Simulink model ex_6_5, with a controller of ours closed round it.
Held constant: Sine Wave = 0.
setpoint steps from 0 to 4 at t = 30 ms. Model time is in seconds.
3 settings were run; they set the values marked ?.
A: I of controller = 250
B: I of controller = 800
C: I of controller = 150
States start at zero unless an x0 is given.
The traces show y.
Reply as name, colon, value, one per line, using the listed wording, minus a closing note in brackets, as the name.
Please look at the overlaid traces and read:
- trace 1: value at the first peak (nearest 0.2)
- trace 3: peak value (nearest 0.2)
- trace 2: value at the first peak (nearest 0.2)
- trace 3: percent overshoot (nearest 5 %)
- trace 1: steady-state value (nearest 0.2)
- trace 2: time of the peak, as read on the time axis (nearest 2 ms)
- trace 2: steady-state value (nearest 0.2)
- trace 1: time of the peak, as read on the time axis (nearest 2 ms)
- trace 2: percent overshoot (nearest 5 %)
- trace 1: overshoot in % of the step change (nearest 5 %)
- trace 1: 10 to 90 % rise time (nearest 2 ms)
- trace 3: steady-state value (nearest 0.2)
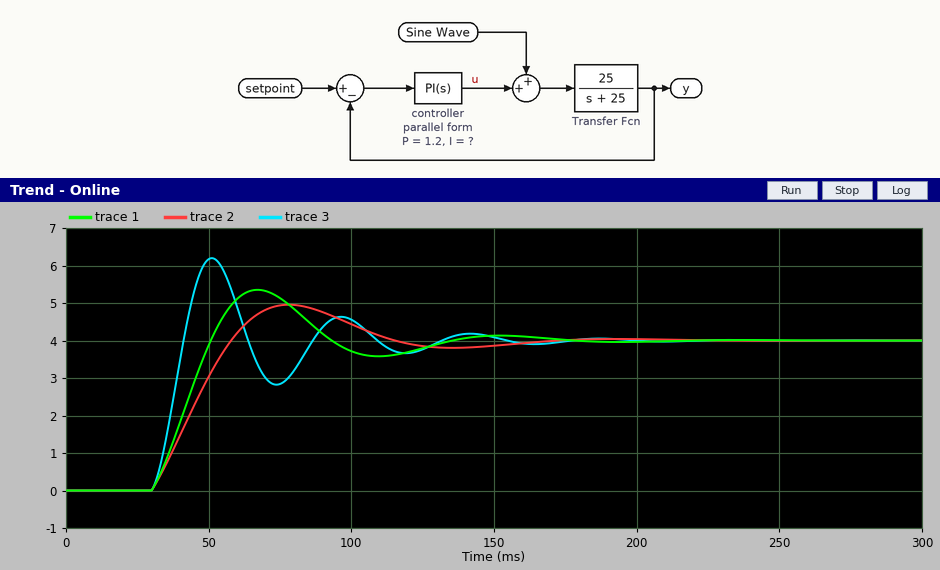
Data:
trace 1: value at the first peak: 5.4
trace 3: peak value: 6.2
trace 2: value at the first peak: 5.0
trace 3: percent overshoot: 55 %
trace 1: steady-state value: 4.0
trace 2: time of the peak, as read on the time axis: 78 ms
trace 2: steady-state value: 4.0
trace 1: time of the peak, as read on the time axis: 68 ms
trace 2: percent overshoot: 25 %
trace 1: overshoot in % of the step change: 35 %
trace 1: 10 to 90 % rise time: 16 ms
trace 3: steady-state value: 4.0
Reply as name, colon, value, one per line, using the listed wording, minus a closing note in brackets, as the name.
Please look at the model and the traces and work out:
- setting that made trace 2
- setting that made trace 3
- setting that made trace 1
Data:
setting that made trace 2: C
setting that made trace 3: B
setting that made trace 1: A
